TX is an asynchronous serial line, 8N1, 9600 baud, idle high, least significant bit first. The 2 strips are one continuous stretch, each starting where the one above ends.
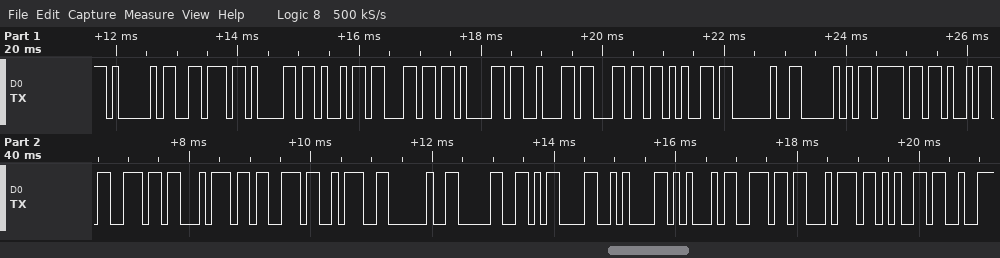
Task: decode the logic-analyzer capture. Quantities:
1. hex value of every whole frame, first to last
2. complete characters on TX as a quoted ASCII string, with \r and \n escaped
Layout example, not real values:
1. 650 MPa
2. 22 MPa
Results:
1. 41 76 61 69 6C 61 62 6C 65 20 50 6F 69 6E 74 73 3A 20 30 0D 0A 45 6E 74 65
2. "Available Points: 0\r\nEnte"
